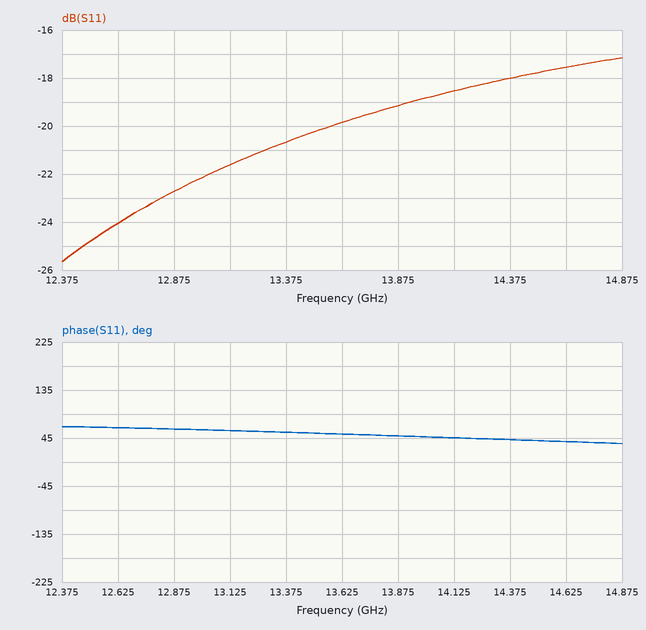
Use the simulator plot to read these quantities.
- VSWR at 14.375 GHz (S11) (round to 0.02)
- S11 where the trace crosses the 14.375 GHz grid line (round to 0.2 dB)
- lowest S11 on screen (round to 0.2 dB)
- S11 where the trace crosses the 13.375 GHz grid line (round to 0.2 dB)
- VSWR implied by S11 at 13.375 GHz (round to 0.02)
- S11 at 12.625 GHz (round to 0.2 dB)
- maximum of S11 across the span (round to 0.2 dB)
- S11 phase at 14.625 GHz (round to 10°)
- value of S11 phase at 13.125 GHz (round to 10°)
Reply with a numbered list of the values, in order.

1. 1.28
2. -18.0 dB
3. -25.6 dB
4. -20.6 dB
5. 1.20
6. -24.0 dB
7. -17.2 dB
8. 40°
9. 60°
